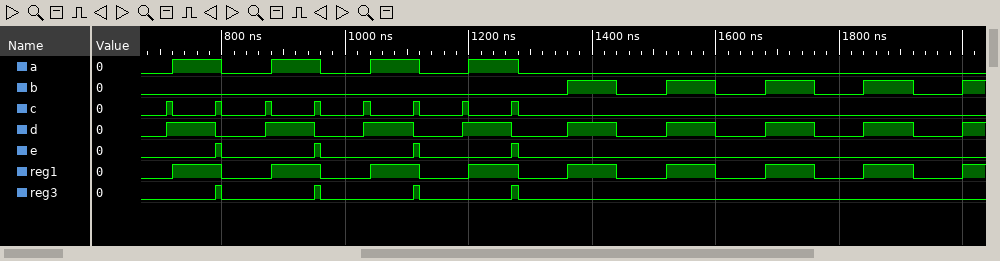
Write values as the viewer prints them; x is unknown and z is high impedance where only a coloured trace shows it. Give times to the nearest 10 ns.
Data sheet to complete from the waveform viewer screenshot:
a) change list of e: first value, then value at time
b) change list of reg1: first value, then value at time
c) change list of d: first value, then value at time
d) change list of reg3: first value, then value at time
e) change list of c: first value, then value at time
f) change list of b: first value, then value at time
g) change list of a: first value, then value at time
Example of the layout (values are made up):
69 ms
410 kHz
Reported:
0, 1 at 790 ns, 0 at 800 ns, 1 at 950 ns, 0 at 960 ns, 1 at 1110 ns, 0 at 1120 ns, 1 at 1270 ns, 0 at 1280 ns
0, 1 at 720 ns, 0 at 800 ns, 1 at 880 ns, 0 at 960 ns, 1 at 1040 ns, 0 at 1120 ns, 1 at 1200 ns, 0 at 1280 ns, 1 at 1360 ns, 0 at 1440 ns, 1 at 1520 ns, 0 at 1600 ns, 1 at 1680 ns, 0 at 1760 ns, 1 at 1840 ns, 0 at 1920 ns, 1 at 2000 ns
0, 1 at 710 ns, 0 at 790 ns, 1 at 870 ns, 0 at 950 ns, 1 at 1030 ns, 0 at 1110 ns, 1 at 1190 ns, 0 at 1270 ns, 1 at 1360 ns, 0 at 1440 ns, 1 at 1520 ns, 0 at 1600 ns, 1 at 1680 ns, 0 at 1760 ns, 1 at 1840 ns, 0 at 1920 ns, 1 at 2000 ns
0, 1 at 790 ns, 0 at 800 ns, 1 at 950 ns, 0 at 960 ns, 1 at 1110 ns, 0 at 1120 ns, 1 at 1270 ns, 0 at 1280 ns
0, 1 at 710 ns, 0 at 720 ns, 1 at 790 ns, 0 at 800 ns, 1 at 870 ns, 0 at 880 ns, 1 at 950 ns, 0 at 960 ns, 1 at 1030 ns, 0 at 1040 ns, 1 at 1110 ns, 0 at 1120 ns, 1 at 1190 ns, 0 at 1200 ns, 1 at 1270 ns, 0 at 1280 ns
0, 1 at 1360 ns, 0 at 1440 ns, 1 at 1520 ns, 0 at 1600 ns, 1 at 1680 ns, 0 at 1760 ns, 1 at 1840 ns, 0 at 1920 ns, 1 at 2000 ns
0, 1 at 720 ns, 0 at 800 ns, 1 at 880 ns, 0 at 960 ns, 1 at 1040 ns, 0 at 1120 ns, 1 at 1200 ns, 0 at 1280 ns
